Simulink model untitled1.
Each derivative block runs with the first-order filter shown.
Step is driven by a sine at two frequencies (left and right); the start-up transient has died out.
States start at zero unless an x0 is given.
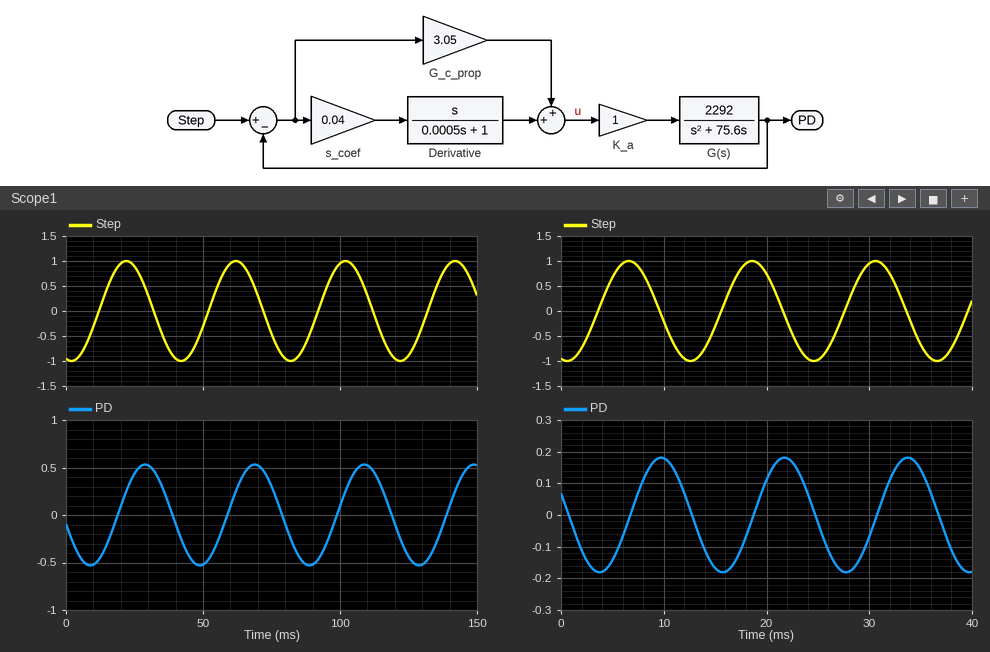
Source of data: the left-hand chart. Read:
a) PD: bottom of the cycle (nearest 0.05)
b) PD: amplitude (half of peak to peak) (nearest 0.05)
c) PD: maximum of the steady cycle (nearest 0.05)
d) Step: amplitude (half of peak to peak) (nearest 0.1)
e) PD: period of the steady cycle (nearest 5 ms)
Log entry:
-0.55
0.55
0.55
1.0
40 ms
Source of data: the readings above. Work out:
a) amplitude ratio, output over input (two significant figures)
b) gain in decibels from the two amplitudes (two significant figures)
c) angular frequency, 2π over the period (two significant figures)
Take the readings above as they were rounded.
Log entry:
0.55
-5.2 dB
0.16 rad/ms
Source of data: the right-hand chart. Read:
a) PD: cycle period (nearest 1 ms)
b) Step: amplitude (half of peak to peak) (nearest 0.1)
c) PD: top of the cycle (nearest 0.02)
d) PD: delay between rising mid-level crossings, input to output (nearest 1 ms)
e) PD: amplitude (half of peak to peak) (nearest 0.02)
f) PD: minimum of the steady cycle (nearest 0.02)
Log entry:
12 ms
1.0
0.18
3 ms
0.18
-0.18
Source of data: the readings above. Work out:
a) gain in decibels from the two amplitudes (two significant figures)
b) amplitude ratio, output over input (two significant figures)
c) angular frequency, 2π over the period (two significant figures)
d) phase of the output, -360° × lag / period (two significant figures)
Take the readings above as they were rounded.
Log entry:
-15 dB
0.18
0.52 rad/ms
-90°
